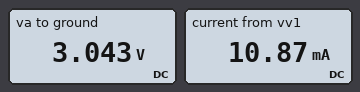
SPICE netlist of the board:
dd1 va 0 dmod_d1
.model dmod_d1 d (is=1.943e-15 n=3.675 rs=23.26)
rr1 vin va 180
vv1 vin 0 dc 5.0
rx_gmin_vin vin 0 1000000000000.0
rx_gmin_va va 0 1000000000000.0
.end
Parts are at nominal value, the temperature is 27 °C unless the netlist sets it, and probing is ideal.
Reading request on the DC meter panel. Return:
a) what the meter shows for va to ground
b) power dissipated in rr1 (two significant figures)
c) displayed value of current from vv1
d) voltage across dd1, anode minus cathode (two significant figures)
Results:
3.043 V
21 mW
10.87 mA
3.0 V
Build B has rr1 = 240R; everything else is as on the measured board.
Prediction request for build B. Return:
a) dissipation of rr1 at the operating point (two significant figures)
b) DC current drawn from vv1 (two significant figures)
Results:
17 mW
8.5 mA
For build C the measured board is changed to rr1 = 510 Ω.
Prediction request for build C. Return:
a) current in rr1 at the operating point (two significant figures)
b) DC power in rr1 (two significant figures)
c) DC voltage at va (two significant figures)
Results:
4.3 mA
9.5 mW
2.8 V
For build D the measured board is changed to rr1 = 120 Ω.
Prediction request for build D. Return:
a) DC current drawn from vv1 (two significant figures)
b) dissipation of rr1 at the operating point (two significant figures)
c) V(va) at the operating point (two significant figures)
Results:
15 mA
28 mW
3.2 V
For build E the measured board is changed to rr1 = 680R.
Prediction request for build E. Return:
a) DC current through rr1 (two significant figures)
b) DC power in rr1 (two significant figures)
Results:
3.3 mA
7.4 mW
